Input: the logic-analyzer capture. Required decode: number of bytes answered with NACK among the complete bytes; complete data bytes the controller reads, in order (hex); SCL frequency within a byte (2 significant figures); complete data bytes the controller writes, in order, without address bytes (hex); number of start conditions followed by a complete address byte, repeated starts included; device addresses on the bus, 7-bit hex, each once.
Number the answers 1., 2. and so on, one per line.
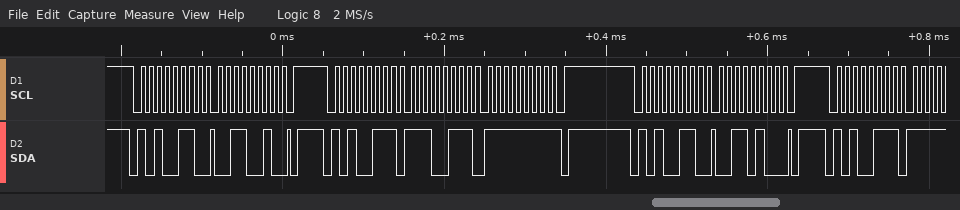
1. 1
2. E7 FF
3. 100 kHz
4. 32 34
5. 4
6. 0x53
